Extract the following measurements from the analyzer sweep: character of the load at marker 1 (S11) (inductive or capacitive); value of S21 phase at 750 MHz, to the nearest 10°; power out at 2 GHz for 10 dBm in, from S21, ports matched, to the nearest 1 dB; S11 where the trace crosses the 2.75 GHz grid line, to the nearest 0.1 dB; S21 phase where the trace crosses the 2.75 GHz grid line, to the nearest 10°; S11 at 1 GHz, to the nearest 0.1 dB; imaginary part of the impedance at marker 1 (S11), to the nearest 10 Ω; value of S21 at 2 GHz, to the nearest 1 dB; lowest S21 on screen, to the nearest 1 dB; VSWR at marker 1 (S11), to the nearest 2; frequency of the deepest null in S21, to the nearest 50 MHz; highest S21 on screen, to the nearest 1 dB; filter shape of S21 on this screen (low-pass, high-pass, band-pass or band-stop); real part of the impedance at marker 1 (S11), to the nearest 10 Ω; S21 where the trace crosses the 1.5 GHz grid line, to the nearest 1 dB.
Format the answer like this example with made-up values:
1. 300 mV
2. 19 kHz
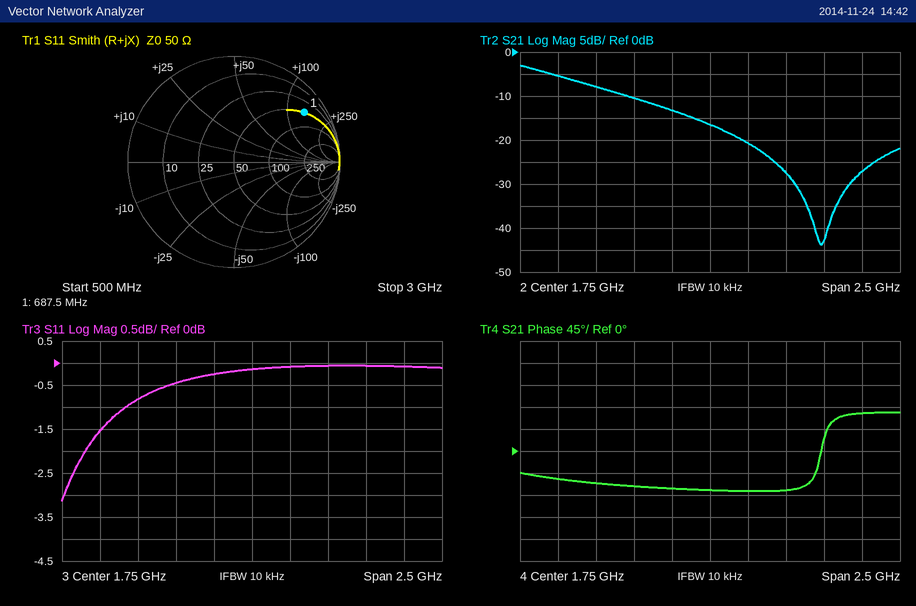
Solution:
1. inductive
2. -60°
3. -11 dBm
4. -0.1 dB
5. 80°
6. -0.8 dB
7. +140 Ω
8. -21 dB
9. -44 dB
10. 10
11. 2.50 GHz
12. -3 dB
13. low-pass
14. 50 Ω
15. -13 dB
